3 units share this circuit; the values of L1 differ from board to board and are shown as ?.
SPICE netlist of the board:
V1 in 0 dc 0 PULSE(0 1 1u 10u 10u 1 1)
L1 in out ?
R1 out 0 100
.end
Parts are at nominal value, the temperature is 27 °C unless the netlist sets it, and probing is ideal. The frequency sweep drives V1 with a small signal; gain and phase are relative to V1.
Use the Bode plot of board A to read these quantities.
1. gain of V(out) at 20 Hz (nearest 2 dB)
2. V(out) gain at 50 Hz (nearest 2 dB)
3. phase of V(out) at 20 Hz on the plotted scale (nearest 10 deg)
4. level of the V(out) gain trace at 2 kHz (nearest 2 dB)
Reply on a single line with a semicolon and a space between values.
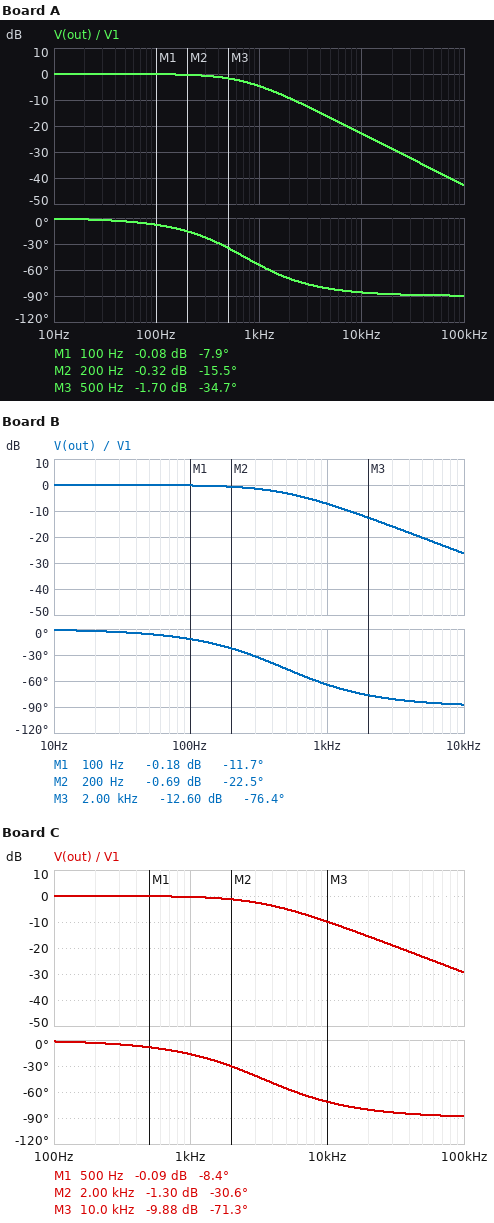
0 dB; 0 dB; 0 deg; -10 dB
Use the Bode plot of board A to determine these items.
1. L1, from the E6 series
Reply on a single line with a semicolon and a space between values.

22 mH
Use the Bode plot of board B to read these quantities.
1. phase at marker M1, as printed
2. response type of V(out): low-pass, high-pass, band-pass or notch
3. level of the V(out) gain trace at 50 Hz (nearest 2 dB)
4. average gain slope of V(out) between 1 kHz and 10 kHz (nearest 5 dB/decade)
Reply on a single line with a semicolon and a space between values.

-11.7 deg; low-pass; 0 dB; -20 dB/decade
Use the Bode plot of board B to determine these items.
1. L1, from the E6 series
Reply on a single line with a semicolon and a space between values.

33 mH
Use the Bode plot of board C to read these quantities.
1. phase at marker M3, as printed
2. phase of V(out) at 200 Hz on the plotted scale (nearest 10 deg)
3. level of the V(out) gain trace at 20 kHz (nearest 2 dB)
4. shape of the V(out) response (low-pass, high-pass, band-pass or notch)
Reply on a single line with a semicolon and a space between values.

-71.3 deg; 0 deg; -16 dB; low-pass
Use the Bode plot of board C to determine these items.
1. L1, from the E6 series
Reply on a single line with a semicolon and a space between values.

4.7 mH
